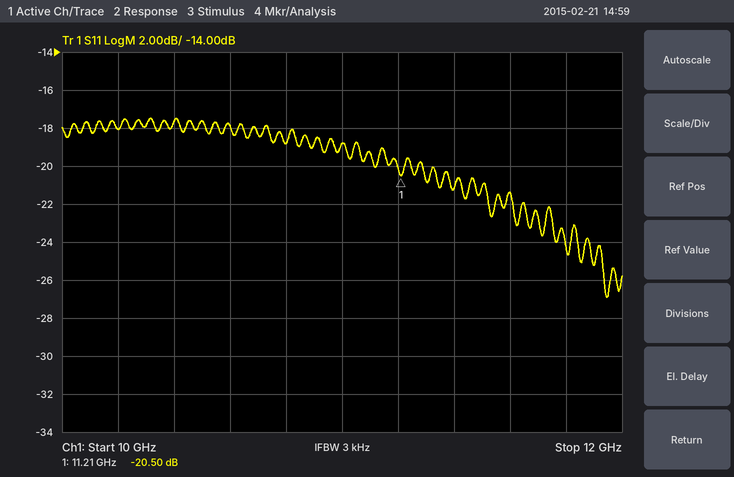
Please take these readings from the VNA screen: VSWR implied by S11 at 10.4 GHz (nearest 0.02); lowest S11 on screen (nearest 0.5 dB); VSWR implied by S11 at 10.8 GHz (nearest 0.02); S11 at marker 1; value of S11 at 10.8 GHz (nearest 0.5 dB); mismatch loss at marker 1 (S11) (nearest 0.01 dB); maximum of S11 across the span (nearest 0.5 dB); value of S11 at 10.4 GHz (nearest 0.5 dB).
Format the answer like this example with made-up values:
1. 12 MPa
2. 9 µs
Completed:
1. 1.30
2. -27.0 dB
3. 1.26
4. -20.50 dB
5. -19.0 dB
6. 0.04 dB
7. -17.5 dB
8. -17.5 dB
